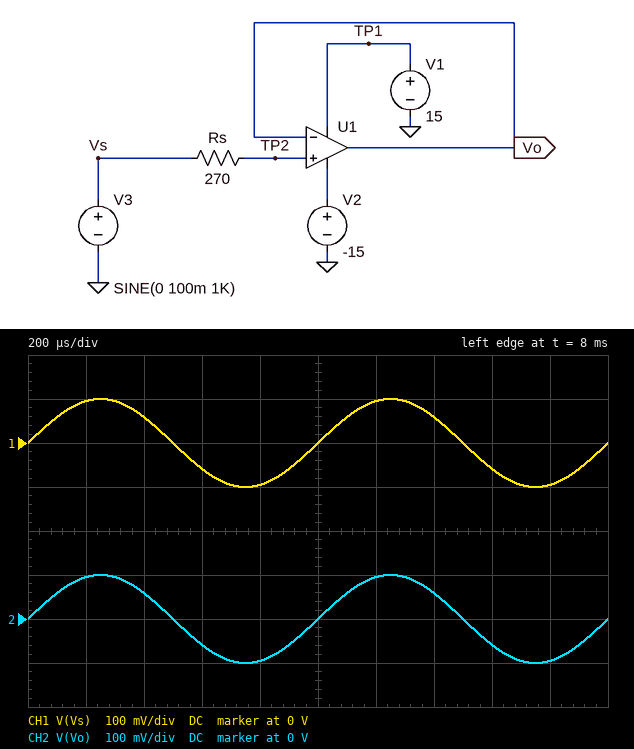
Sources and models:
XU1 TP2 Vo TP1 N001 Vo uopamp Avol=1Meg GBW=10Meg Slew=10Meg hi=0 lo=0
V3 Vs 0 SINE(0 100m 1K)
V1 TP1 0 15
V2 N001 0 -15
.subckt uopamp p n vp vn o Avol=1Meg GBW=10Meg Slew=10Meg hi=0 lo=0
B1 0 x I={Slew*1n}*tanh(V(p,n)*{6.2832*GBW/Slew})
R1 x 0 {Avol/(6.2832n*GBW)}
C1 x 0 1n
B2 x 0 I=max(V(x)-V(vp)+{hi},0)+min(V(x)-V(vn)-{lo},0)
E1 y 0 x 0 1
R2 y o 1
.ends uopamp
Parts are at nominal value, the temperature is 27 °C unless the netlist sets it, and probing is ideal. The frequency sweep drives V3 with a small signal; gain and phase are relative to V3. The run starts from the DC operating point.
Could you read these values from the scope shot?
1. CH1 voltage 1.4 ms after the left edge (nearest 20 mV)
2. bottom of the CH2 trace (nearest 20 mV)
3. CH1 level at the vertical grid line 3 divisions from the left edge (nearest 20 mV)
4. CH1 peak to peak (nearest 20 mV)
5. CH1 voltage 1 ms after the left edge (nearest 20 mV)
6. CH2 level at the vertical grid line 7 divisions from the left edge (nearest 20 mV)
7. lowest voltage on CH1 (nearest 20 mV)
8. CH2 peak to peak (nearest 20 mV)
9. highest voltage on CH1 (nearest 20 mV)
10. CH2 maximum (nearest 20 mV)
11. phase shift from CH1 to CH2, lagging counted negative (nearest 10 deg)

60 mV
-100 mV
-60 mV
200 mV
0 V
60 mV
-100 mV
200 mV
100 mV
100 mV
0 deg
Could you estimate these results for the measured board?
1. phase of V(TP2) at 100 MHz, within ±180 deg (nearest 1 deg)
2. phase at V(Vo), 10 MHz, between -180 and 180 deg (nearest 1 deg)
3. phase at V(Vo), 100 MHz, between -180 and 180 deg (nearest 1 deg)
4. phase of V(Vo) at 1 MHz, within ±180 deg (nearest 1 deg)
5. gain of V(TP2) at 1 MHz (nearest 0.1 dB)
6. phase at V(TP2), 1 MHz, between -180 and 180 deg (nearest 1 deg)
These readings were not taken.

0 deg
-45 deg
-84 deg
-6 deg
0 dB
0 deg
